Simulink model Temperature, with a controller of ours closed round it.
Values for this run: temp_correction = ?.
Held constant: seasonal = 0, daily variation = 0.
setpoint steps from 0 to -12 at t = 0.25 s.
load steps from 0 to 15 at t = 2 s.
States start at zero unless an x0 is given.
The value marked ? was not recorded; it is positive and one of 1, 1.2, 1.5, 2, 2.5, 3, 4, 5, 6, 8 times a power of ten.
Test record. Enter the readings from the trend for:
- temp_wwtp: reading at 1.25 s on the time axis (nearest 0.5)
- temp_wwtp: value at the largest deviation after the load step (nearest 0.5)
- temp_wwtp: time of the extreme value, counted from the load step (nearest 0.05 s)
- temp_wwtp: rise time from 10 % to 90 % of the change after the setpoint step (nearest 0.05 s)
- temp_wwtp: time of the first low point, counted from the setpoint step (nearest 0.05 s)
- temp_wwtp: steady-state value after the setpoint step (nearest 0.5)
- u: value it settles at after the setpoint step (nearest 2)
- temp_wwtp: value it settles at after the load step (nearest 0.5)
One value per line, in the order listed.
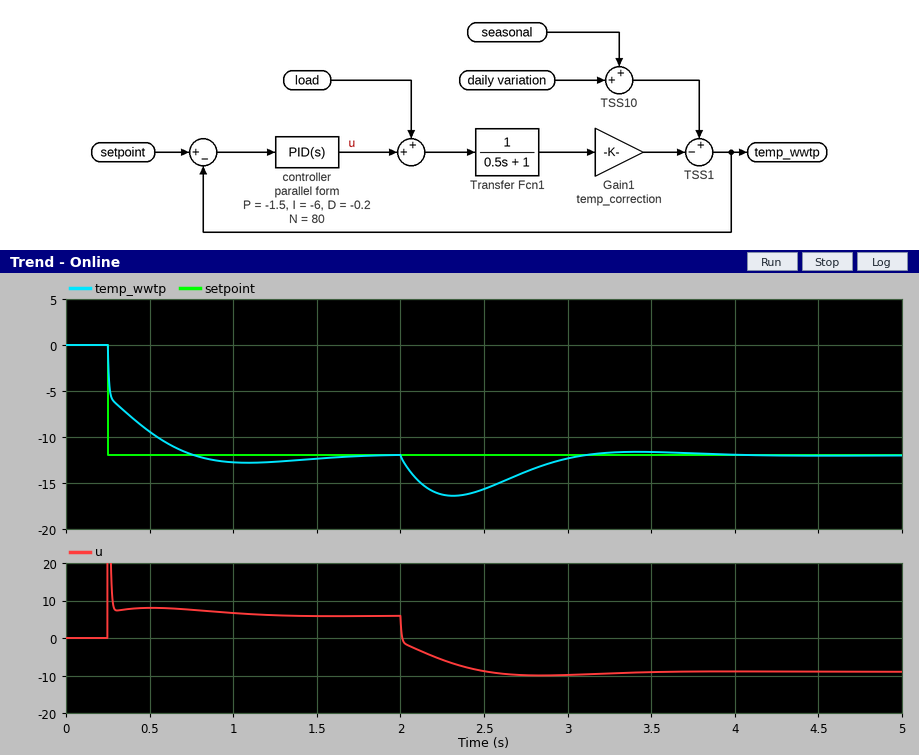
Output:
-12.5
-16.5
0.30 s
0.35 s
0.85 s
-12.0
6
-12.0
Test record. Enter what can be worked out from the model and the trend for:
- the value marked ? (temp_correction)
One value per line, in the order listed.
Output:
2
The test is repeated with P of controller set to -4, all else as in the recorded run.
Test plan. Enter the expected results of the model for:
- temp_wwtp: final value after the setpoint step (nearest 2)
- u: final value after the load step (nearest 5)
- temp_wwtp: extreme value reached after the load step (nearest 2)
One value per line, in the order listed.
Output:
-12
-10
-14
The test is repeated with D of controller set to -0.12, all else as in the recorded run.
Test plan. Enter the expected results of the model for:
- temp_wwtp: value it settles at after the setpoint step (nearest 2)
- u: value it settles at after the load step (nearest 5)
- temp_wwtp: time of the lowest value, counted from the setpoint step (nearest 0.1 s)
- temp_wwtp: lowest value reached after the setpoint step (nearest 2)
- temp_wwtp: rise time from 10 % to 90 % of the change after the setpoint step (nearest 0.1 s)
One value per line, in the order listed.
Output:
-12
-10
0.7 s
-12
0.3 s
